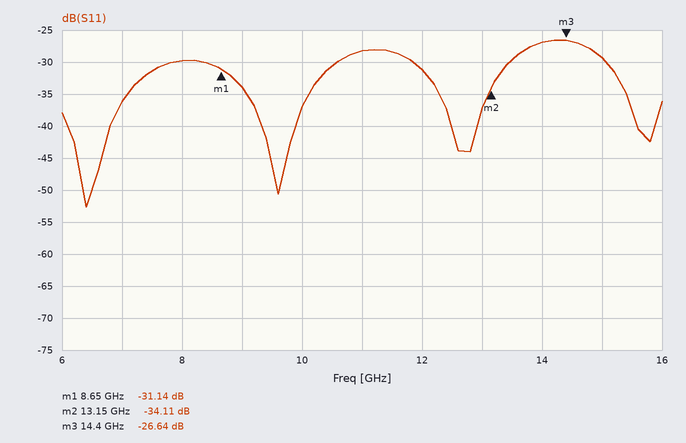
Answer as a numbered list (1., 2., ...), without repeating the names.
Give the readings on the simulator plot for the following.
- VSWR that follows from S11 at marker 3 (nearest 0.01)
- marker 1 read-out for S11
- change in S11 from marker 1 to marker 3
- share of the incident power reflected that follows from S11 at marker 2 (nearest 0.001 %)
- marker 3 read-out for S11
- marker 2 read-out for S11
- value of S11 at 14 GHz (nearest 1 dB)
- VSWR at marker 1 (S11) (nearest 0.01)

1. 1.10
2. -31.14 dB
3. 4.50 dB
4. 0.039 %
5. -26.64 dB
6. -34.11 dB
7. -27 dB
8. 1.06
